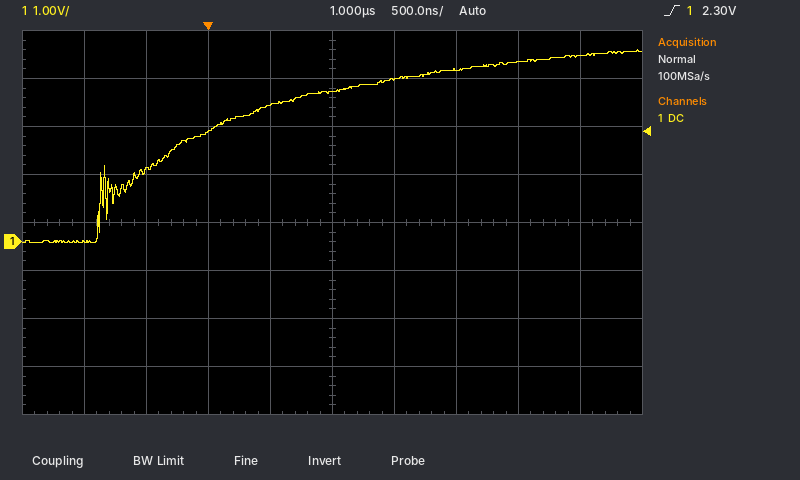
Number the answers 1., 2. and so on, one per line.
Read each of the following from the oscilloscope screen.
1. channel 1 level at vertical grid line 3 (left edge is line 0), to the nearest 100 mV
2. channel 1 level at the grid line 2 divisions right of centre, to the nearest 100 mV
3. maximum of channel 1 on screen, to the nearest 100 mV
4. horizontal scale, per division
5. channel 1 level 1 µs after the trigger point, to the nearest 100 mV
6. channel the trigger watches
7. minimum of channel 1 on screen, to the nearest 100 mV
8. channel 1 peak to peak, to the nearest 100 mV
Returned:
1. 2.3 V
2. 3.6 V
3. 4.0 V
4. 500 ns
5. 3.1 V
6. channel 1
7. 0.0 V
8. 4.0 V
